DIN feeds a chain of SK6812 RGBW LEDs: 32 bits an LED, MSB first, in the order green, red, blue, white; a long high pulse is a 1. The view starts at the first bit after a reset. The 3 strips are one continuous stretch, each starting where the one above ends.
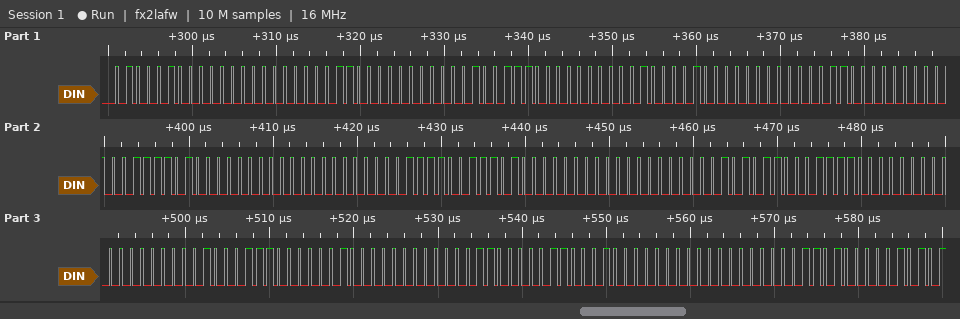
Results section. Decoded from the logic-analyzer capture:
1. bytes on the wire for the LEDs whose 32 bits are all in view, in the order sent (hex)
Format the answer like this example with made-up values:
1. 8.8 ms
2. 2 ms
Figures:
1. 44 00 06 00 27 00 21 00 0C 00 3D 00 00 0F 3A 00 00 2B 1E 00 00 47 02 00 18 31 00 00
